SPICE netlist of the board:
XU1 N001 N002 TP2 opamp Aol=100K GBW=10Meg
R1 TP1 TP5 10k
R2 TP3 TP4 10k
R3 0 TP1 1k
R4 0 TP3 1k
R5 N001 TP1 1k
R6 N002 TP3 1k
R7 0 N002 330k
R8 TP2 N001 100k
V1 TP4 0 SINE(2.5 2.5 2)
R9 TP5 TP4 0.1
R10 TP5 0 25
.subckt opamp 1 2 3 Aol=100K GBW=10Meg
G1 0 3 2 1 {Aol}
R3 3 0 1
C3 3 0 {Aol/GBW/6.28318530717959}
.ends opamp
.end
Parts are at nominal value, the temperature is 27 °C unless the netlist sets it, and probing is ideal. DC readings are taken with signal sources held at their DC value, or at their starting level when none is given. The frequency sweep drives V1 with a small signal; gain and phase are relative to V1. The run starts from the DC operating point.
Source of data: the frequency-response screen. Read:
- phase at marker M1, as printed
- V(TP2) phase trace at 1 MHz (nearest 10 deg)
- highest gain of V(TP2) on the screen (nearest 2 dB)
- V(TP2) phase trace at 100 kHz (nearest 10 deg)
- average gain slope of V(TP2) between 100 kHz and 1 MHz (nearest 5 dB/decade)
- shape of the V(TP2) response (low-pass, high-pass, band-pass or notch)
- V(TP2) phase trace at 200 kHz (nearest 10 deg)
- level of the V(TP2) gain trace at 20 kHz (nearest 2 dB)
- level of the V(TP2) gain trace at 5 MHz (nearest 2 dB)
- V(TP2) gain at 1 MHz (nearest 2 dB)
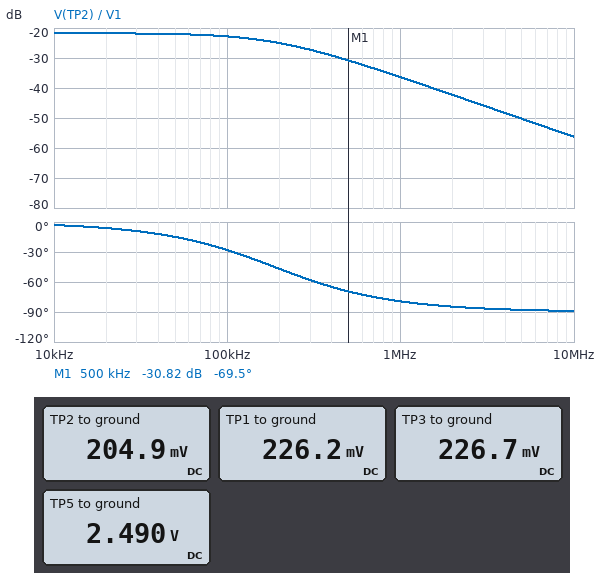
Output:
-69.5 deg
-80 deg
-22 dB
-30 deg
-15 dB/decade
low-pass
-50 deg
-22 dB
-50 dB
-36 dB
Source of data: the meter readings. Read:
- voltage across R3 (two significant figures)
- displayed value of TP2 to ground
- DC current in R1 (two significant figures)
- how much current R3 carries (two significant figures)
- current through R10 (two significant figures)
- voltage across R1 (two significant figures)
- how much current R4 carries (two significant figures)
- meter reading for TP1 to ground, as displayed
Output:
230 mV
204.9 mV
230 µA
230 µA
100 mA
2.3 V
230 µA
226.2 mV
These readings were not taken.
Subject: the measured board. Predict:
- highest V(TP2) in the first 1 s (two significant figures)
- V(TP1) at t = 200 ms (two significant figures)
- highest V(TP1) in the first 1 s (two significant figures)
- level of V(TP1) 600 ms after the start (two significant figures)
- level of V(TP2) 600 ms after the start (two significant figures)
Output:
410 mV
360 mV
450 mV
440 mV
400 mV
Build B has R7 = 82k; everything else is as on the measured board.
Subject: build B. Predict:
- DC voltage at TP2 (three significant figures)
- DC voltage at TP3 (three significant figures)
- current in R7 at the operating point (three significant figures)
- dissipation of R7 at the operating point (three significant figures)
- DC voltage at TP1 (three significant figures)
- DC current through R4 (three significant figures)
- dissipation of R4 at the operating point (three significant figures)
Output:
-1.22 mV
225 mV
2.71 µA
602 nW
224 mV
225 µA
50.5 µW
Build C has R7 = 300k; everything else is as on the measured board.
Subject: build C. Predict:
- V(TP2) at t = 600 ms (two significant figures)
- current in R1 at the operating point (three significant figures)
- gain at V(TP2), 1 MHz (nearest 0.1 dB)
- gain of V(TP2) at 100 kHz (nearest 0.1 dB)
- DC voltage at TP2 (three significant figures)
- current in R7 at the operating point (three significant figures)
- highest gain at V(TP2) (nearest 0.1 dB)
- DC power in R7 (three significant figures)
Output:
390 mV
226 µA
-36.7 dB
-23.1 dB
198 mV
753 nA
-22.0 dB
170 nW
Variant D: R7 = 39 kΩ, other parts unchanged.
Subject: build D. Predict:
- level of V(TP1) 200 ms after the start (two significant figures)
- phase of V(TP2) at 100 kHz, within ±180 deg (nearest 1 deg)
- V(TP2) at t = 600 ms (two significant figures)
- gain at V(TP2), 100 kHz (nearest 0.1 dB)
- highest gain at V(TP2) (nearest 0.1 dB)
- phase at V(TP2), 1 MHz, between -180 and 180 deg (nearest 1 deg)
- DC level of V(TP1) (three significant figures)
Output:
350 mV
152 deg
-570 mV
-19.8 dB
-18.7 dB
101 deg
222 mV
